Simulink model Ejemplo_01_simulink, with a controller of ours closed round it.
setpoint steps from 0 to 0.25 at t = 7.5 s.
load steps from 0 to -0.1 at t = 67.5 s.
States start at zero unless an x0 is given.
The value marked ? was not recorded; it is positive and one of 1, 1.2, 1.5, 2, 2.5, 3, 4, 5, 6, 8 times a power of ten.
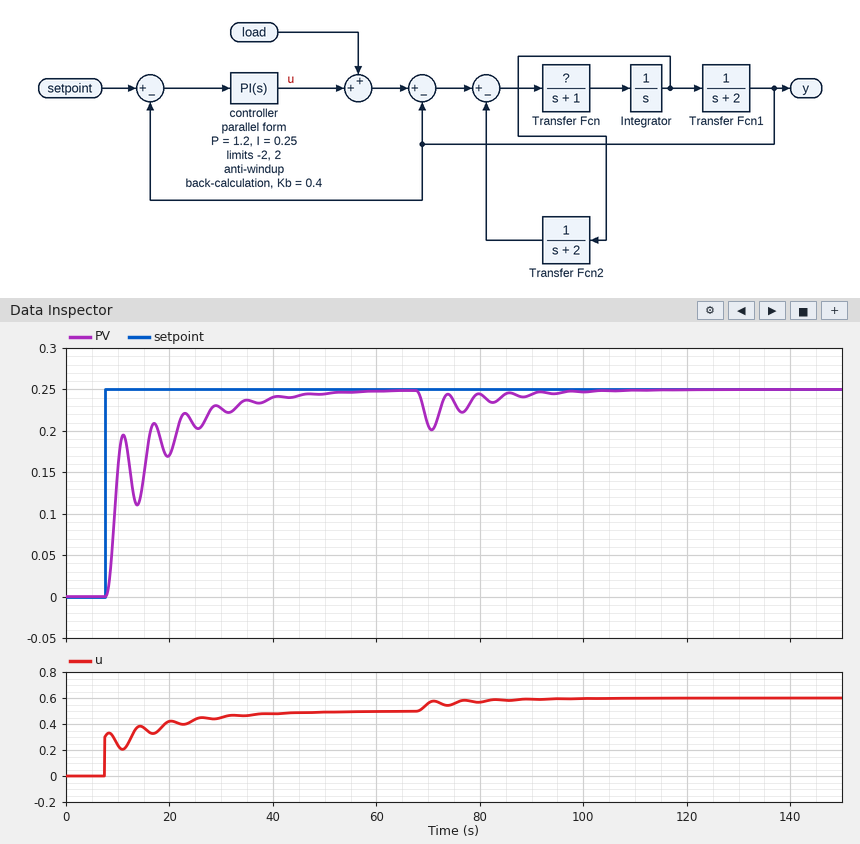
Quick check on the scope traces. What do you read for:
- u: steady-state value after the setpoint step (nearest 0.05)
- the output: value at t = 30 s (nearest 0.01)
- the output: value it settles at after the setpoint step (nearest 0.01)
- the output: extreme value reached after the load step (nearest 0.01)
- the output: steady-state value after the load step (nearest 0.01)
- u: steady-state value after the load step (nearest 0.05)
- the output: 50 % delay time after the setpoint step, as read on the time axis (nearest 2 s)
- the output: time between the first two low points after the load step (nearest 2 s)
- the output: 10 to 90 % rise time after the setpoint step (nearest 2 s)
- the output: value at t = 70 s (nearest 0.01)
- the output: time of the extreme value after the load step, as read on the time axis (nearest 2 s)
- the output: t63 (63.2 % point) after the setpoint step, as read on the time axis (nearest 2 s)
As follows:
0.50
0.23
0.25
0.20
0.25
0.60
10 s
6 s
20 s
0.21
70 s
10 s
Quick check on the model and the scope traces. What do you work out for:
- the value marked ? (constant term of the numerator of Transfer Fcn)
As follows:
1
